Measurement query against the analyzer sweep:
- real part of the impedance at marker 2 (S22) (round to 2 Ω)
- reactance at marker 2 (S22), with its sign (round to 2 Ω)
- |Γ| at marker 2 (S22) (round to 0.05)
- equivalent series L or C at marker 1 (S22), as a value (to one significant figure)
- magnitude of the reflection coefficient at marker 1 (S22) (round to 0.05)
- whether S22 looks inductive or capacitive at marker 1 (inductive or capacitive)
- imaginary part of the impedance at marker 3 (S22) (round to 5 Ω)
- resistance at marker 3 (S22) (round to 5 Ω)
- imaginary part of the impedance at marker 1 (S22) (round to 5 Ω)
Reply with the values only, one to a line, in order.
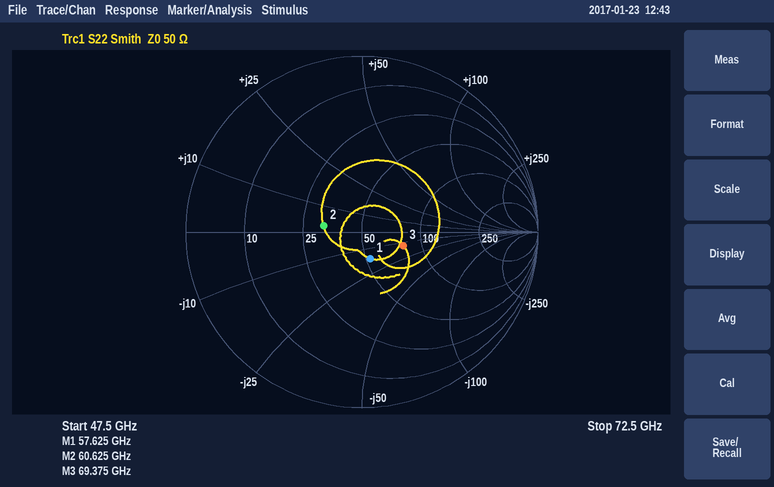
32 Ω
+2 Ω
0.20
200 fF
0.15
capacitive
-15 Ω
80 Ω
-15 Ω
